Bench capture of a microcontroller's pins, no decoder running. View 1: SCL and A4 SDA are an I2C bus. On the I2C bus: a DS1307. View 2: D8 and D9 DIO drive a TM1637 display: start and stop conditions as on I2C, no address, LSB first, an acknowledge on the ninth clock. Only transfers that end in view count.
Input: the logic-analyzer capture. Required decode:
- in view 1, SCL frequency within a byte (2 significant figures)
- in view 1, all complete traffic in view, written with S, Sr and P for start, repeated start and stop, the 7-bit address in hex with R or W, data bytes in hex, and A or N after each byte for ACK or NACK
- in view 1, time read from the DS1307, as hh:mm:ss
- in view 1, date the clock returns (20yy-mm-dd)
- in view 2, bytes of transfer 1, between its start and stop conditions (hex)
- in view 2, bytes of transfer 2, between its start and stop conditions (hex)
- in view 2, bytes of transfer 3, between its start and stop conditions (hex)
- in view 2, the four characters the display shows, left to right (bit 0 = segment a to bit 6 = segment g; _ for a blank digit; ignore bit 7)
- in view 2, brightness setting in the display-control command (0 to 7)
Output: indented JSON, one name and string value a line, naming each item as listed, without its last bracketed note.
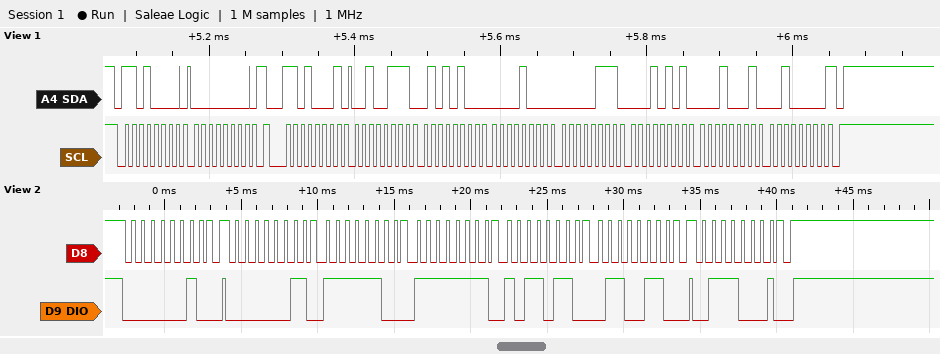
{
  "in view 1, SCL frequency within a byte": "100 kHz",
  "in view 1, all complete traffic in view, written with S, Sr and P for start, repeated start and stop, the 7-bit address in hex with R or W, data bytes in hex, and A or N after each byte for ACK or NACK": "S 68W A 00 A Sr 68R A 27 A 54 A 08 A 07 A 15 A 11 A 20 N P",
  "in view 1, time read from the DS1307, as hh:mm:ss": "08:54:27",
  "in view 1, date the clock returns": "2020-11-15",
  "in view 2, bytes of transfer 1, between its start and stop conditions": "40",
  "in view 2, bytes of transfer 2, between its start and stop conditions": "C0 3F FF 6D 66",
  "in view 2, bytes of transfer 3, between its start and stop conditions": "8E",
  "in view 2, the four characters the display shows, left to right": "0854",
  "in view 2, brightness setting in the display-control command": "6"
}
